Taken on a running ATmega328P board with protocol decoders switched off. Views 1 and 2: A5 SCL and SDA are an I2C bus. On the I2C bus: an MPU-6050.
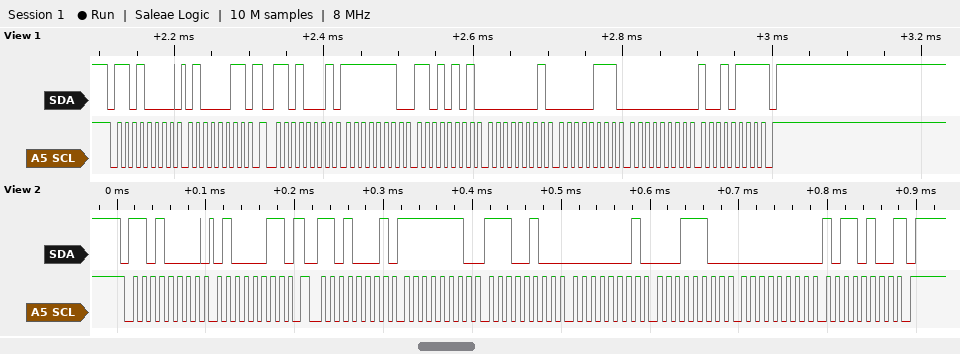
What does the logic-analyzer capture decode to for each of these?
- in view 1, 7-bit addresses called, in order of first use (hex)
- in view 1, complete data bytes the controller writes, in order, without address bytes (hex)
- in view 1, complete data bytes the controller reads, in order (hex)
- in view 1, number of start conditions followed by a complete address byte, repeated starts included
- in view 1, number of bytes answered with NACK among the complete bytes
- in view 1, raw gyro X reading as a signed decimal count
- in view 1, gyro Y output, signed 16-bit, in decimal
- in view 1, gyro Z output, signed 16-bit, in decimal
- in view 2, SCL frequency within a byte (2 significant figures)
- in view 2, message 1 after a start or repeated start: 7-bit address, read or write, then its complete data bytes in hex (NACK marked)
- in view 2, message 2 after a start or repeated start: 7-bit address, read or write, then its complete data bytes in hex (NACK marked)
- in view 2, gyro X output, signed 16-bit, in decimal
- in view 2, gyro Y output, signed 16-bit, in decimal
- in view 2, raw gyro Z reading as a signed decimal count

0x68
43
FE D5 01 07 00 97
2
1
-299
263
151
100 kHz
0x68 write: 43
0x68 read: FE E4 01 1C 00 B4 NACK
-284
284
180
